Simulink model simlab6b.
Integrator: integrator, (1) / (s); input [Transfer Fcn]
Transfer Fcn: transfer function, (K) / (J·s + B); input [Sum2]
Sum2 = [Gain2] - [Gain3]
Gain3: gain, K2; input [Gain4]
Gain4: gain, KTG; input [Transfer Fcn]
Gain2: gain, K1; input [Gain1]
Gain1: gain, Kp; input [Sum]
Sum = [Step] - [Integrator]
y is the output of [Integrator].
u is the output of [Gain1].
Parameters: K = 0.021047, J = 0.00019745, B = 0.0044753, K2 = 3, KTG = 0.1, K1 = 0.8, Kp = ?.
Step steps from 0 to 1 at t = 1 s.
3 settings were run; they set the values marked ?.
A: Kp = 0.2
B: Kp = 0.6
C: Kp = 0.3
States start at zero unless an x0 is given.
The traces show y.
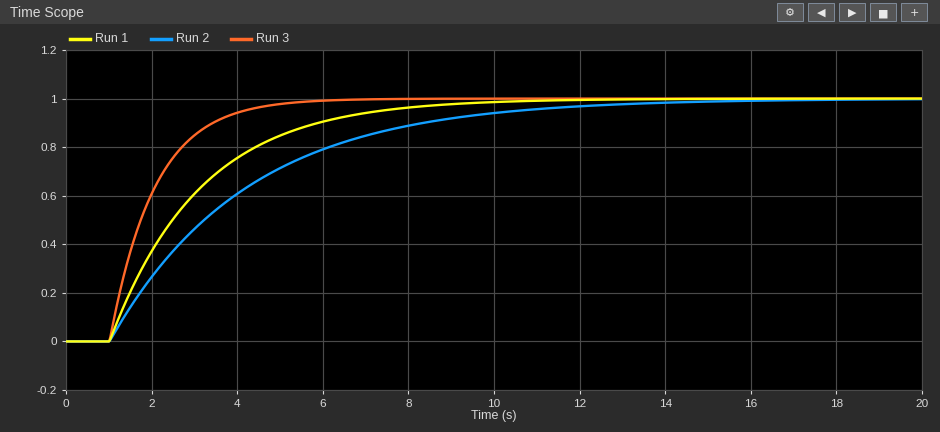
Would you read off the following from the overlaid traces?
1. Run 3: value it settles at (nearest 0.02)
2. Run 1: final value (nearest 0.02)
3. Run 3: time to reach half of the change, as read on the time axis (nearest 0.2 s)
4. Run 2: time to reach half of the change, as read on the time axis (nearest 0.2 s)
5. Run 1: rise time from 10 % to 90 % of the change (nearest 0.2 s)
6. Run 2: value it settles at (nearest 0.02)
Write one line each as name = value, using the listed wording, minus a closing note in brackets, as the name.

Run 3: value it settles at = 1.00
Run 1: final value = 1.00
Run 3: time to reach half of the change, as read on the time axis = 1.8 s
Run 2: time to reach half of the change, as read on the time axis = 3.2 s
Run 1: rise time from 10 % to 90 % of the change = 4.6 s
Run 2: value it settles at = 1.00
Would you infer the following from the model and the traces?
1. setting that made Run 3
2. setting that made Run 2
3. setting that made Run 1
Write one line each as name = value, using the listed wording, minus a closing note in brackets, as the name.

setting that made Run 3 = B
setting that made Run 2 = A
setting that made Run 1 = C
